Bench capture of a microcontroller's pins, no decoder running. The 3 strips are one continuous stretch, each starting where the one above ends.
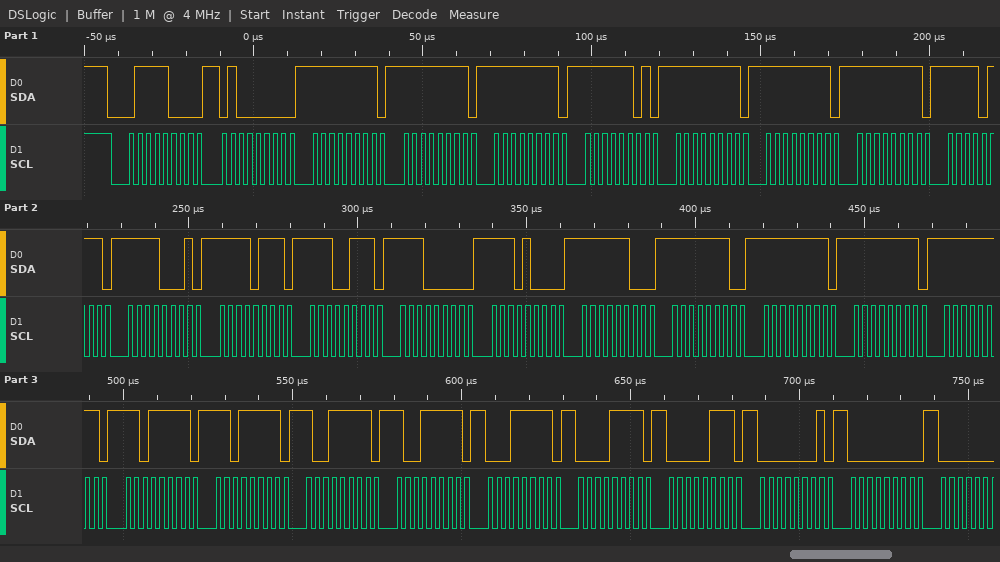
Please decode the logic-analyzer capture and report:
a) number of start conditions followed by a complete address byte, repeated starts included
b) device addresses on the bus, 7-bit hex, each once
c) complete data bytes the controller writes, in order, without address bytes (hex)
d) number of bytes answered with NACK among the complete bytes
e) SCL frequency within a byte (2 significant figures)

1
0x3C
40 FF FF FF FD FF FF FF F7 F1 F7 E7 E0 E8 FC FE FF FF FF DF DF 9F 9F 1F 0F 07 01 00
0
400 kHz
